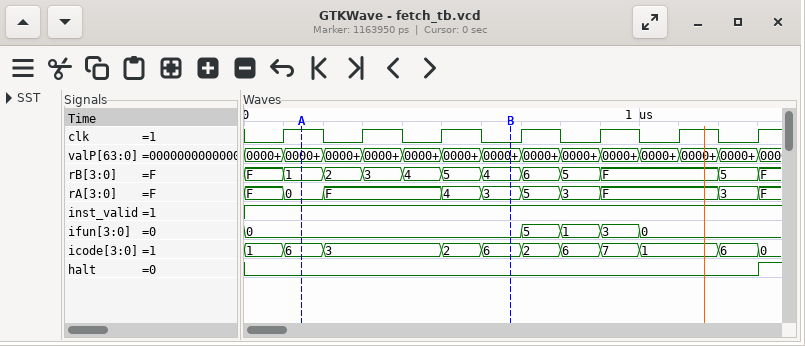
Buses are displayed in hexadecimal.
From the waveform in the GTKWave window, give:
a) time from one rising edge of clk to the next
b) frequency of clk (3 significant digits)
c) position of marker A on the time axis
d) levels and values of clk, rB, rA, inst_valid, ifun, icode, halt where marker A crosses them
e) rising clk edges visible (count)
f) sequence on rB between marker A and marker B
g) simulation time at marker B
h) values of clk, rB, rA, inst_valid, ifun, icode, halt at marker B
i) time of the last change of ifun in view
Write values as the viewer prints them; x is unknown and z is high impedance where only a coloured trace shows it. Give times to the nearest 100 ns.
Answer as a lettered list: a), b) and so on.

a) 200 ns
b) 5.00 MHz
c) 100 ns
d) clk=1, rB=1, rA=0, inst_valid=1, ifun=0, icode=6, halt=0
e) 7
f) 1, 2, 3, 4, 5, 4
g) 700 ns
h) clk=0, rB=4, rA=3, inst_valid=1, ifun=0, icode=6, halt=0
i) 1000 ns
